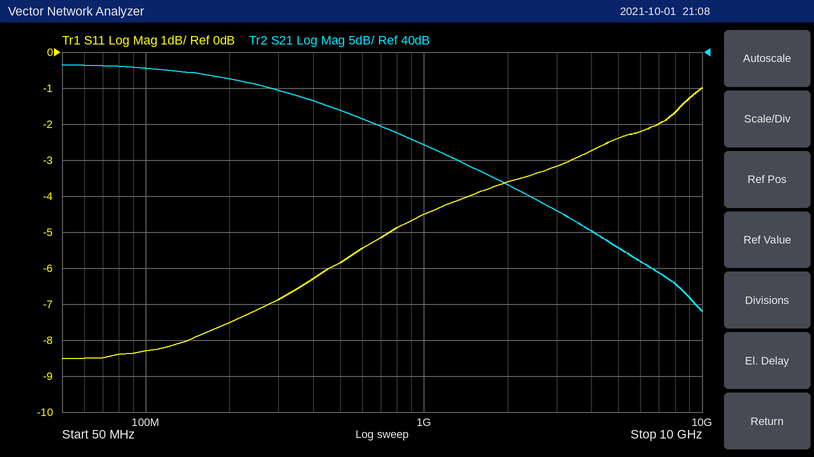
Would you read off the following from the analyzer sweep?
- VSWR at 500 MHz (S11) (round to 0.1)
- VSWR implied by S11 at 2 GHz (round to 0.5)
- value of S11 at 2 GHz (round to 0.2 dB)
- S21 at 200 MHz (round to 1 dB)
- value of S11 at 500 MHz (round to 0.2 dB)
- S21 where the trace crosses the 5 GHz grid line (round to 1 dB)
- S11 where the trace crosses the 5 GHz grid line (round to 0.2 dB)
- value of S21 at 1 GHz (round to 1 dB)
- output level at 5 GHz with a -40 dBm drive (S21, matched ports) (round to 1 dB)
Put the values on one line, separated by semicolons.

3.1; 5.0; -3.6 dB; 36 dB; -5.8 dB; 13 dB; -2.4 dB; 27 dB; -27 dBm
